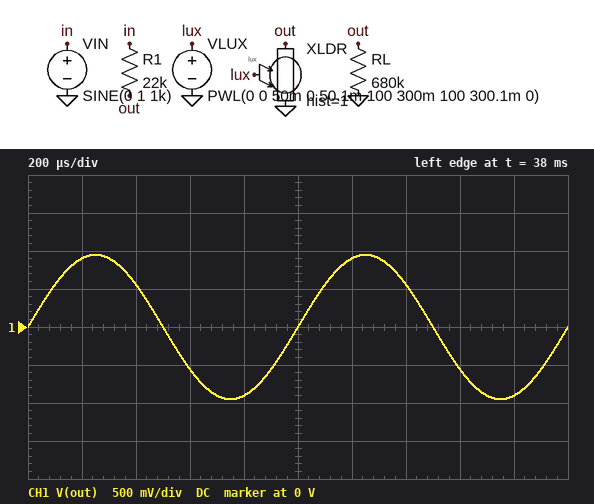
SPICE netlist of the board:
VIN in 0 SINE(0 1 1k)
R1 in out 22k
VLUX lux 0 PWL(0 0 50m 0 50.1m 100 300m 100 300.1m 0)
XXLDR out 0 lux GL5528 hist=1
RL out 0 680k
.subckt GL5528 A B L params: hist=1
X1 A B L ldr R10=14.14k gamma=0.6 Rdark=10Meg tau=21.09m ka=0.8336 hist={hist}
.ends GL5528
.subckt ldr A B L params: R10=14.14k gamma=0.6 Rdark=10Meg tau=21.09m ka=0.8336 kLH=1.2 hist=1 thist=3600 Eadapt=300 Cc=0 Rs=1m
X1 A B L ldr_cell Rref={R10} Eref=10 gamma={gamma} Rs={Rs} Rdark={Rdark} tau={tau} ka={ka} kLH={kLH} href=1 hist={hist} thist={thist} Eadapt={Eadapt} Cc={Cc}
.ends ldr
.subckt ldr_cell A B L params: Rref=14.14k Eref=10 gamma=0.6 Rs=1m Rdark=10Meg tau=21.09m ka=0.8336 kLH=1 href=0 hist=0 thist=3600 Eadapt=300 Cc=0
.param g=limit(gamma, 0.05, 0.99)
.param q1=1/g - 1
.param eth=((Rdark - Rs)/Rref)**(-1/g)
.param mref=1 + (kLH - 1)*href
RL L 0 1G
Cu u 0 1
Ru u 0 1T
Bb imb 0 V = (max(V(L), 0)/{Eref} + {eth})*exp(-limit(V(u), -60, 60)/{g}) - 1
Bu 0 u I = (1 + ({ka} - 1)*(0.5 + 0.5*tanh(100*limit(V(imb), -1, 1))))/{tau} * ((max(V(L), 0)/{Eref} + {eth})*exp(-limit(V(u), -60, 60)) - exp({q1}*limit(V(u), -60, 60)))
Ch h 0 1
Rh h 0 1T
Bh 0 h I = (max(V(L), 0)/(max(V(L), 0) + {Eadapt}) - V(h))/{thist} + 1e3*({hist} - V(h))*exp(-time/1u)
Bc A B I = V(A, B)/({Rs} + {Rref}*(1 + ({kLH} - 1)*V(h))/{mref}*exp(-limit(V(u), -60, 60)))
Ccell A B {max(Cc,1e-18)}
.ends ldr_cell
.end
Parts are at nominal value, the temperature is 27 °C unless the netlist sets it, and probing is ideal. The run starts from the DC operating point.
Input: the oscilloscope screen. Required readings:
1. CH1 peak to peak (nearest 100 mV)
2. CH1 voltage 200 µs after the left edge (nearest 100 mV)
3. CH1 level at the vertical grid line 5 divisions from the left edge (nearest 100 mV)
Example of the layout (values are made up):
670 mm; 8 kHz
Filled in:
1.9 V; 900 mV; 0 V
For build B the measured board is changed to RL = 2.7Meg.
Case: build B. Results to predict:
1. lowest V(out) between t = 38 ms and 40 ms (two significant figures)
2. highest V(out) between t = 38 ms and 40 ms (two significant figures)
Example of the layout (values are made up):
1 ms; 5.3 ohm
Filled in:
-970 mV; 970 mV
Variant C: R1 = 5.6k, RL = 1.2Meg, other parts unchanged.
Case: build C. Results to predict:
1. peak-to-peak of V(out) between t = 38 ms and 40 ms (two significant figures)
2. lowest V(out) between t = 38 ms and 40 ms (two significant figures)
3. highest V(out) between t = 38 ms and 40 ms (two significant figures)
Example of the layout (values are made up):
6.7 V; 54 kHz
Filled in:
2.0 V; -990 mV; 990 mV
